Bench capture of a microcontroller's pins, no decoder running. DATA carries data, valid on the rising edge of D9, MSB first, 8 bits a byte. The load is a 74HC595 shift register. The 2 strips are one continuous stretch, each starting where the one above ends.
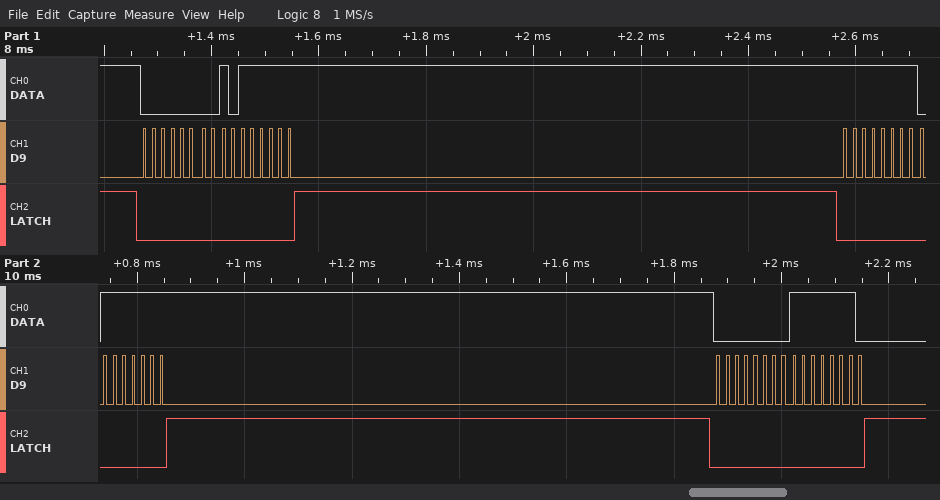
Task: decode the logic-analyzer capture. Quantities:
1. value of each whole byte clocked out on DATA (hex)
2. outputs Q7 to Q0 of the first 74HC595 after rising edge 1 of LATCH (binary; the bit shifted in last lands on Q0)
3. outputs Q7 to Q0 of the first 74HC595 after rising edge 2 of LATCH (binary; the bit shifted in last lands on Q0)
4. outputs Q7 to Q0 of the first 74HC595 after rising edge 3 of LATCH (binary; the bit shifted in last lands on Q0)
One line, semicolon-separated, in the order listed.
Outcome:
00 BF FF 7F 00 FE; 10111111; 01111111; 11111110
